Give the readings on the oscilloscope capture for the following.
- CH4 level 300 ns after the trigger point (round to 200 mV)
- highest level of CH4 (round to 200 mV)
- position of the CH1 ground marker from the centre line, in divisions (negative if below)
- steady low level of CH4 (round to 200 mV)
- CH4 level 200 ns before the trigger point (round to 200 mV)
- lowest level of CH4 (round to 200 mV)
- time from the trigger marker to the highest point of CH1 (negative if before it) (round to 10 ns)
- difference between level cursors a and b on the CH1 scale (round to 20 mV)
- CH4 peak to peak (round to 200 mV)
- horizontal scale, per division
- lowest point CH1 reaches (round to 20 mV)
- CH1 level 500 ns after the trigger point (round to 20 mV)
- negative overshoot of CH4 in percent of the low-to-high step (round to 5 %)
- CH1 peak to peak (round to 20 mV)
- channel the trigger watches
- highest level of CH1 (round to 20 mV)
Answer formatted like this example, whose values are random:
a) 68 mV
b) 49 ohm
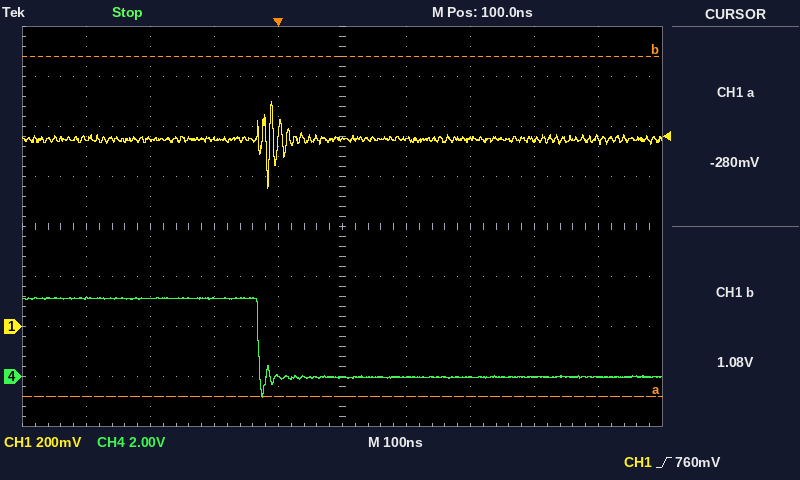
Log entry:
a) 0.0 V
b) 3.2 V
c) -2.0 div
d) 0.0 V
e) 3.2 V
f) -800 mV
g) -10 ns
h) 1.36 V
i) 4.0 V
j) 100 ns
k) 560 mV
l) 740 mV
m) 25 %
n) 340 mV
o) CH1
p) 900 mV
